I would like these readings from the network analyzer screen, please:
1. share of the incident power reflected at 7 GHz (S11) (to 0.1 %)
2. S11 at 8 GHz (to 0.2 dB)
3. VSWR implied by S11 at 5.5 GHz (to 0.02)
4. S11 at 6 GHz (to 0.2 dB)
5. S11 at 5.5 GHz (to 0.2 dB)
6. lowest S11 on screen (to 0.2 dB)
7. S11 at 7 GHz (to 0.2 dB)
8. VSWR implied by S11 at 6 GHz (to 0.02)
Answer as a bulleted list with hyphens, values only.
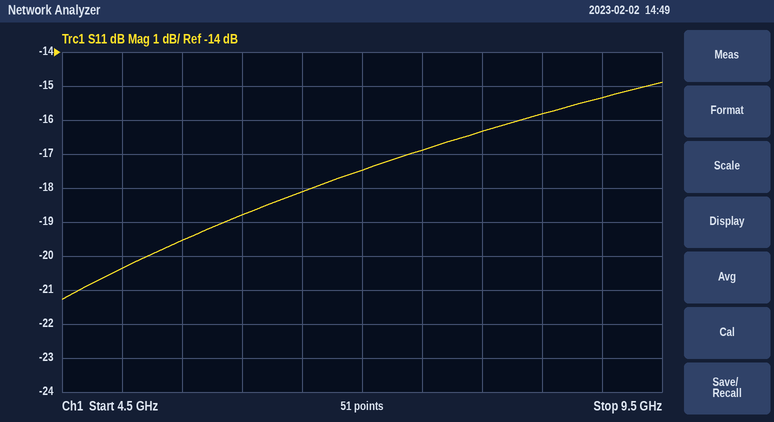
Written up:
- 1.8 %
- -16.4 dB
- 1.24
- -18.8 dB
- -19.6 dB
- -21.2 dB
- -17.4 dB
- 1.26
